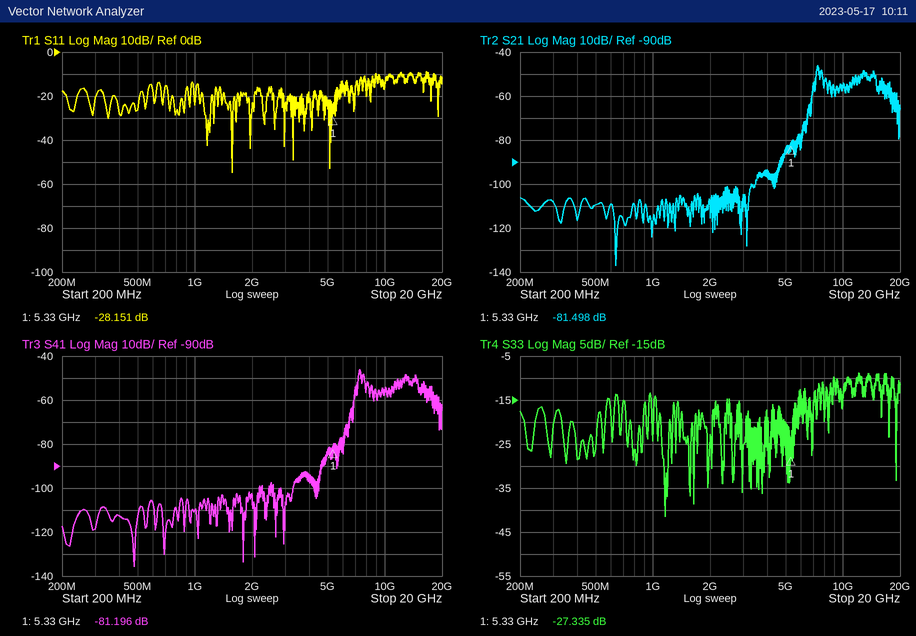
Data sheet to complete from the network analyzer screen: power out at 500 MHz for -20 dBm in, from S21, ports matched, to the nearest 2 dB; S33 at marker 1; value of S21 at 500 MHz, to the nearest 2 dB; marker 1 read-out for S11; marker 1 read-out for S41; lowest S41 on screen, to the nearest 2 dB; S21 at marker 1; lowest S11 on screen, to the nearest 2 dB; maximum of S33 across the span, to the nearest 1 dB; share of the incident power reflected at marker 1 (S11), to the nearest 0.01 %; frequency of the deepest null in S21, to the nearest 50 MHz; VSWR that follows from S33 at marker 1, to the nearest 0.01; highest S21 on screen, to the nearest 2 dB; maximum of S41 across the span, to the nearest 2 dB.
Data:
-130 dBm
-27.335 dB
-110 dB
-28.151 dB
-81.196 dB
-136 dB
-81.498 dB
-54 dB
-9 dB
0.15 %
650 MHz
1.09
-46 dB
-46 dB
